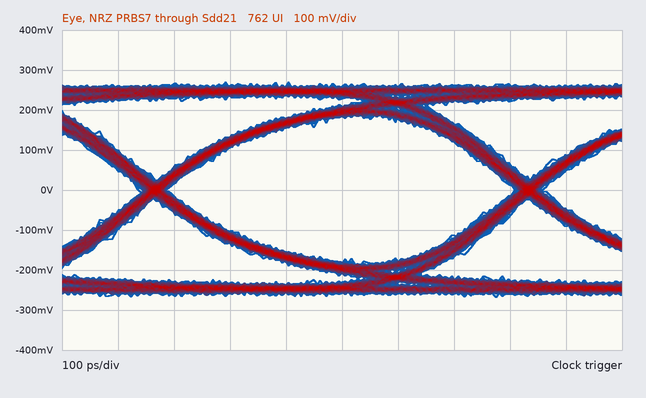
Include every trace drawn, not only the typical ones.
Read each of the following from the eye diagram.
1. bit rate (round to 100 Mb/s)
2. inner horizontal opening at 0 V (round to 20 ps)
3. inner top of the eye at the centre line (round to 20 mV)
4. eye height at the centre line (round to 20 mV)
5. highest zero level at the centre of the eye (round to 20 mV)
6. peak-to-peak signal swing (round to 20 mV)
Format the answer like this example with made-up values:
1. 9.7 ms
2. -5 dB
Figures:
1. 1.5 Gb/s
2. 620 ps
3. 180 mV
4. 360 mV
5. -180 mV
6. 540 mV
